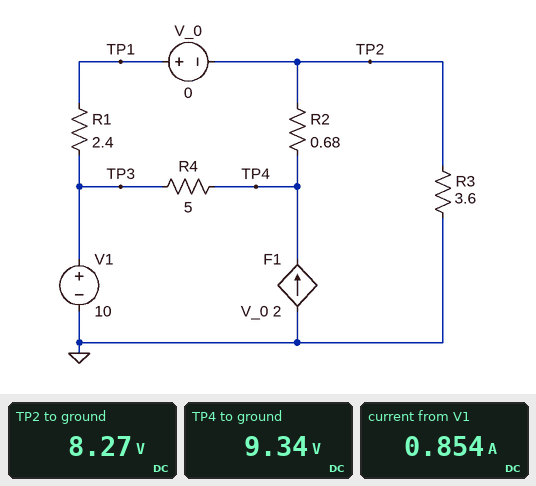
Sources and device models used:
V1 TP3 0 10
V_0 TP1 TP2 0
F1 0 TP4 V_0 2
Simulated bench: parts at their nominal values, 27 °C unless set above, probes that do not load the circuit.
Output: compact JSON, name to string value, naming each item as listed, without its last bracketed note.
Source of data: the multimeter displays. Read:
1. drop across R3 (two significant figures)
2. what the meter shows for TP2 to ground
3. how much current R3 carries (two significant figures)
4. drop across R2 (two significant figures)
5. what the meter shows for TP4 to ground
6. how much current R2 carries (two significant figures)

{"drop across R3": "8.3 V", "what the meter shows for TP2 to ground": "8.27 V", "how much current R3 carries": "2.3 A", "drop across R2": "1.1 V", "what the meter shows for TP4 to ground": "9.34 V", "how much current R2 carries": "1.6 A"}
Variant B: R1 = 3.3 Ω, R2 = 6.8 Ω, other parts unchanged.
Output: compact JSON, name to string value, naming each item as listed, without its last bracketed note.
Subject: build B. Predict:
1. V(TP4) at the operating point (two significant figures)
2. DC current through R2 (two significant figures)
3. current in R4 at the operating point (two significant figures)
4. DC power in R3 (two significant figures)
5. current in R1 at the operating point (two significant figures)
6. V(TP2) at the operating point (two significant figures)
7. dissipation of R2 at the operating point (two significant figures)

{"V(TP4) at the operating point": "14 V", "DC current through R2": "1.0 A", "current in R4 at the operating point": "800 mA", "DC power in R3": "14 W", "current in R1 at the operating point": "910 mA", "V(TP2) at the operating point": "7.0 V", "dissipation of R2 at the operating point": "7.2 W"}
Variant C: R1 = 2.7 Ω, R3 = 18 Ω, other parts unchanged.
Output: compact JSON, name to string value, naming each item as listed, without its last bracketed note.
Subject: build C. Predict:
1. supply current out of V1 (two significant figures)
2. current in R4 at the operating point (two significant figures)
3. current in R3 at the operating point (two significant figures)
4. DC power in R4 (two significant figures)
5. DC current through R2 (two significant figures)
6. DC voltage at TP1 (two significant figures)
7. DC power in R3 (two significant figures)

{"supply current out of V1": "200 mA", "current in R4 at the operating point": "39 mA", "current in R3 at the operating point": "530 mA", "DC power in R4": "7.5 mW", "DC current through R2": "370 mA", "DC voltage at TP1": "9.6 V", "DC power in R3": "5.1 W"}
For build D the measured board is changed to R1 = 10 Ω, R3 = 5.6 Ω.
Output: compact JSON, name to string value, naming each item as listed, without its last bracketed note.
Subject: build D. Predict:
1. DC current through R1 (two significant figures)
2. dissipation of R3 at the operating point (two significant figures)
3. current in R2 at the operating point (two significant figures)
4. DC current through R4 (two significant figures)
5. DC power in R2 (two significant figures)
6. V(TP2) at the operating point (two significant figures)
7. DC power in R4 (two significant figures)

{"DC current through R1": "280 mA", "dissipation of R3 at the operating point": "9.2 W", "current in R2 at the operating point": "1.0 A", "DC current through R4": "430 mA", "DC power in R2": "680 mW", "V(TP2) at the operating point": "7.2 V", "DC power in R4": "930 mW"}
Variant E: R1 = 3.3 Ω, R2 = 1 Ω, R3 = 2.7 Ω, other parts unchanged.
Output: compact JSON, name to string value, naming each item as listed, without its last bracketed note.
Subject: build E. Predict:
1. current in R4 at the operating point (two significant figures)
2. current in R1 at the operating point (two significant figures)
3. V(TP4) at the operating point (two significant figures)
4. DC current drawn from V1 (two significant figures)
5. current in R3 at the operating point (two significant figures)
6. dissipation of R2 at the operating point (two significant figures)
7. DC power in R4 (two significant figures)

{"current in R4 at the operating point": "180 mA", "current in R1 at the operating point": "830 mA", "V(TP4) at the operating point": "9.1 V", "DC current drawn from V1": "1.0 A", "current in R3 at the operating point": "2.7 A", "dissipation of R2 at the operating point": "3.4 W", "DC power in R4": "160 mW"}
